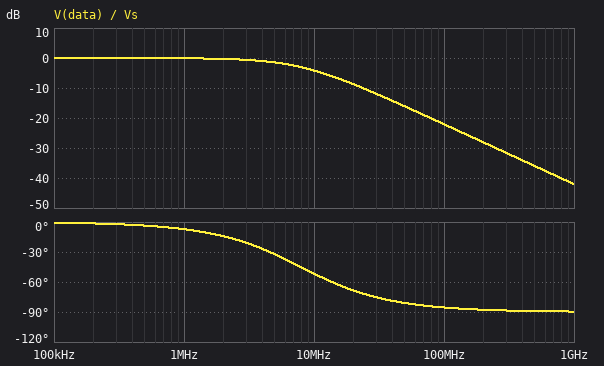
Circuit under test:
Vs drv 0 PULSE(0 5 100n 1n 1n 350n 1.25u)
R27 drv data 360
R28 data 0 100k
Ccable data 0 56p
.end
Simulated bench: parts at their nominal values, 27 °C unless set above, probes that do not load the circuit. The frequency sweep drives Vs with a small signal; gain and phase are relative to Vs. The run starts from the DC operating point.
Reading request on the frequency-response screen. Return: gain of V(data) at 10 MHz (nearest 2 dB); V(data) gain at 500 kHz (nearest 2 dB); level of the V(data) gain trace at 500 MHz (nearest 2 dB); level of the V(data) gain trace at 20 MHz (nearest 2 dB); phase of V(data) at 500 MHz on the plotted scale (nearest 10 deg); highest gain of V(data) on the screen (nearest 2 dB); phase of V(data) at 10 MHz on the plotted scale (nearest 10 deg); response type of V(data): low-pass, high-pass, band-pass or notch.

-4 dB
0 dB
-36 dB
-8 dB
-90 deg
0 dB
-50 deg
low-pass
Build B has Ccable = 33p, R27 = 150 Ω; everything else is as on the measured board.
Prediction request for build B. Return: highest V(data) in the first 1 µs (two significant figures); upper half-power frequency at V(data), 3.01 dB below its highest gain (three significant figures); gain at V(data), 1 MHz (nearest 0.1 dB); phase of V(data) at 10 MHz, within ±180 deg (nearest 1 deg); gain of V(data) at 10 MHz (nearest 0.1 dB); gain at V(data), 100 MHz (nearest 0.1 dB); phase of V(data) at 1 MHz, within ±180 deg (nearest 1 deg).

5.0 V
32.2 MHz
0 dB
-17 deg
-0.4 dB
-10.3 dB
-2 deg
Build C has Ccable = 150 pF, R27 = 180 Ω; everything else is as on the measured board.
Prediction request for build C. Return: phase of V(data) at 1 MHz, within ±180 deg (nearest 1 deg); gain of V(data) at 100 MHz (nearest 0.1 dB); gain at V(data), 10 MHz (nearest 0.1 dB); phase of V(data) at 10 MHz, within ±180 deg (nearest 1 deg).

-10 deg
-24.6 dB
-5.9 dB
-59 deg
